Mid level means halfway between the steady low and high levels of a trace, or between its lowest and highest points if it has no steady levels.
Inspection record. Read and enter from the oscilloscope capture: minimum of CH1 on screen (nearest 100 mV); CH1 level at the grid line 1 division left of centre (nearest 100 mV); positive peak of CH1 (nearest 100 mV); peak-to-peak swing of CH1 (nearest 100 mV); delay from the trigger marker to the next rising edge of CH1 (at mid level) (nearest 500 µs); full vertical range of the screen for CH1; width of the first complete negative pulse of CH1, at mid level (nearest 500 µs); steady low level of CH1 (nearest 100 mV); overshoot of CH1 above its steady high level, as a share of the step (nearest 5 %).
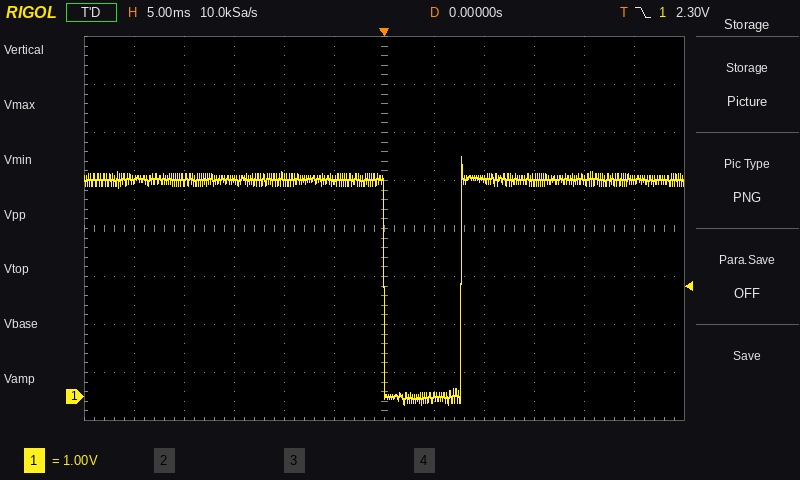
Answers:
-200 mV
4.5 V
5.0 V
5.2 V
7.5 ms
8 V
7.5 ms
0.0 V
10 %
